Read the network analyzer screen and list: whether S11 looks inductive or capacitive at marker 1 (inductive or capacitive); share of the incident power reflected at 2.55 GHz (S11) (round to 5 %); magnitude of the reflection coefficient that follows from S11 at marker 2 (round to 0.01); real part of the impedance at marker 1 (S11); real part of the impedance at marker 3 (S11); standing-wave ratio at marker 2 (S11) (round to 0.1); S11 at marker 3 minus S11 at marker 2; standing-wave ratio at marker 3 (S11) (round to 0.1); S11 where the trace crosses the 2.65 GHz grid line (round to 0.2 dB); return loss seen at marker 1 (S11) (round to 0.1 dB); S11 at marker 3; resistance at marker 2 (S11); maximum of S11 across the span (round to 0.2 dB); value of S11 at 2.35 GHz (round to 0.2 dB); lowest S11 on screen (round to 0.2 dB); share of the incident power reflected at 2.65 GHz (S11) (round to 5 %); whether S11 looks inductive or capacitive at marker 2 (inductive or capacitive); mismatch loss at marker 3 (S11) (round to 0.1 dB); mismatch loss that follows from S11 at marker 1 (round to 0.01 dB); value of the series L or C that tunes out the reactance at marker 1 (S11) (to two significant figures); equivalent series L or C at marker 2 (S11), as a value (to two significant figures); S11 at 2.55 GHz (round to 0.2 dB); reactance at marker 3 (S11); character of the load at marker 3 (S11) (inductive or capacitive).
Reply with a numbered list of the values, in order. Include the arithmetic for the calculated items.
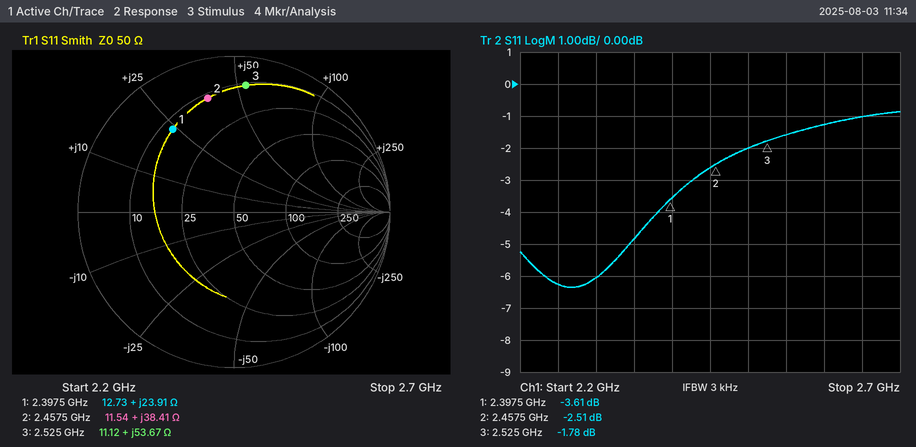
1. inductive
2. 10^(-1.6/10) ≈ 69.2 %, so 70 % to the nearest 5 %
3. 10^(-2.51/20) ≈ 0.75
4. 12.73 Ω
5. 11.12 Ω
6. 7.0
7. -1.78 − (-2.51) = 0.73 dB
8. 9.8
9. -1.0 dB
10. 3.6 dB
11. -1.78 dB
12. 11.54 Ω
13. -0.8 dB
14. -4.8 dB
15. -6.4 dB
16. 10^(-1/10) ≈ 79.4 %, so 80 % to the nearest 5 %
17. inductive
18. −10 log10(1 − 10^(-1.78/10)) ≈ 4.7 dB
19. −10 log10(1 − 10^(-3.61/10)) ≈ 2.48 dB
20. C = 1/(2π × 2.3975 GHz × 23.91 Ω) ≈ 2.8 pF
21. L = 38.41 Ω/(2π × 2.4575 GHz) ≈ 2.5 nH
22. -1.6 dB
23. +53.67 Ω
24. inductive
